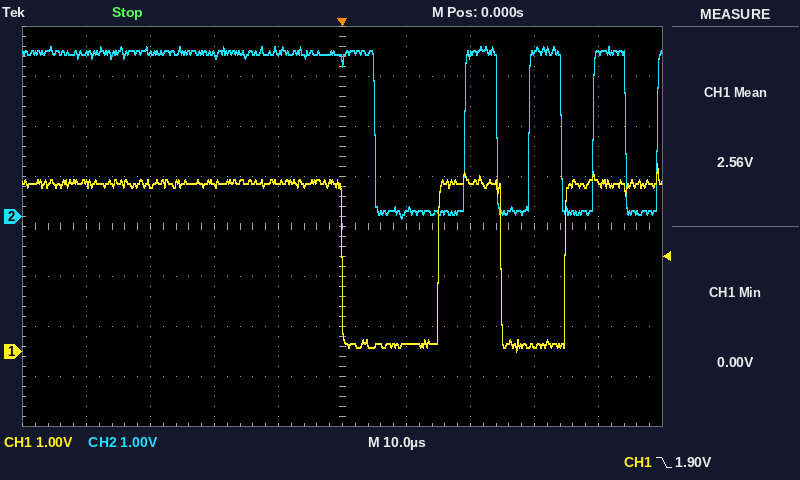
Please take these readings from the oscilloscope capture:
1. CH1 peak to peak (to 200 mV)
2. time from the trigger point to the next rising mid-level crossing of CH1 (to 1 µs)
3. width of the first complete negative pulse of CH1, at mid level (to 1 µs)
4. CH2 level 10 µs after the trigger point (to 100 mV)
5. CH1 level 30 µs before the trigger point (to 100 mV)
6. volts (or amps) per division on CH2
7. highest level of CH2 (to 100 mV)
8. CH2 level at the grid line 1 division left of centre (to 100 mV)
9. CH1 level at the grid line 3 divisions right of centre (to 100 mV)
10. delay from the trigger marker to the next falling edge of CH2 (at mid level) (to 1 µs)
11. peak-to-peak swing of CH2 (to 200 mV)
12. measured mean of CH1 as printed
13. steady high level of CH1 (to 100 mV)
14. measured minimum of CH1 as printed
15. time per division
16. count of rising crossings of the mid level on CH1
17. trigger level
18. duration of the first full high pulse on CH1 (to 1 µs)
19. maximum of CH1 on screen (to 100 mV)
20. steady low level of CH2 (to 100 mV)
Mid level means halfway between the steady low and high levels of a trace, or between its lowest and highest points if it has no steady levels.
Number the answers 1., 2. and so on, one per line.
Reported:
1. 3.8 V
2. 15 µs
3. 15 µs
4. 100 mV
5. 3.4 V
6. 1 V
7. 3.4 V
8. 3.3 V
9. 100 mV
10. 5 µs
11. 3.4 V
12. 2.56 V
13. 3.4 V
14. 0.00 V
15. 10 µs
16. 2
17. 1.90 V
18. 10 µs
19. 3.8 V
20. 100 mV
